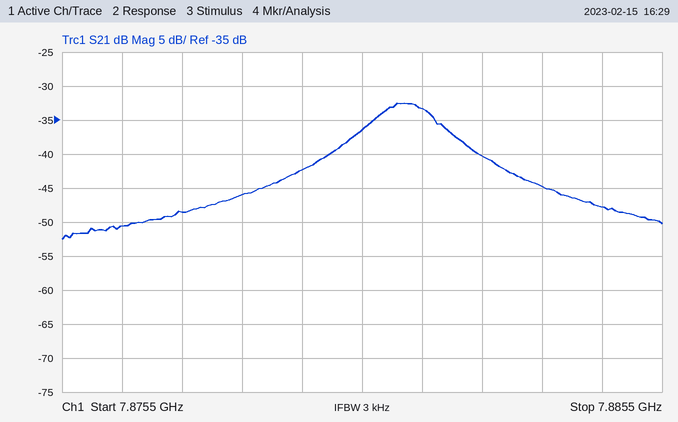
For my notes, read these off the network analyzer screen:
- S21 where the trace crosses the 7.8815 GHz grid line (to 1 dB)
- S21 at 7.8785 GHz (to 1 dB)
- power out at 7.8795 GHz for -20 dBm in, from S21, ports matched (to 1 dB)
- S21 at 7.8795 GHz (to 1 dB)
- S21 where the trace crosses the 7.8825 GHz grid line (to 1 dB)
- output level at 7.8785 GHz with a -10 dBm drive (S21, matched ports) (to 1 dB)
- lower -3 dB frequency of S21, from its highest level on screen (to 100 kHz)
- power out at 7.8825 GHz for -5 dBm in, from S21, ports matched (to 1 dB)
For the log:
-33 dB
-46 dB
-62 dBm
-42 dB
-40 dB
-56 dBm
7.8806 GHz
-45 dBm
